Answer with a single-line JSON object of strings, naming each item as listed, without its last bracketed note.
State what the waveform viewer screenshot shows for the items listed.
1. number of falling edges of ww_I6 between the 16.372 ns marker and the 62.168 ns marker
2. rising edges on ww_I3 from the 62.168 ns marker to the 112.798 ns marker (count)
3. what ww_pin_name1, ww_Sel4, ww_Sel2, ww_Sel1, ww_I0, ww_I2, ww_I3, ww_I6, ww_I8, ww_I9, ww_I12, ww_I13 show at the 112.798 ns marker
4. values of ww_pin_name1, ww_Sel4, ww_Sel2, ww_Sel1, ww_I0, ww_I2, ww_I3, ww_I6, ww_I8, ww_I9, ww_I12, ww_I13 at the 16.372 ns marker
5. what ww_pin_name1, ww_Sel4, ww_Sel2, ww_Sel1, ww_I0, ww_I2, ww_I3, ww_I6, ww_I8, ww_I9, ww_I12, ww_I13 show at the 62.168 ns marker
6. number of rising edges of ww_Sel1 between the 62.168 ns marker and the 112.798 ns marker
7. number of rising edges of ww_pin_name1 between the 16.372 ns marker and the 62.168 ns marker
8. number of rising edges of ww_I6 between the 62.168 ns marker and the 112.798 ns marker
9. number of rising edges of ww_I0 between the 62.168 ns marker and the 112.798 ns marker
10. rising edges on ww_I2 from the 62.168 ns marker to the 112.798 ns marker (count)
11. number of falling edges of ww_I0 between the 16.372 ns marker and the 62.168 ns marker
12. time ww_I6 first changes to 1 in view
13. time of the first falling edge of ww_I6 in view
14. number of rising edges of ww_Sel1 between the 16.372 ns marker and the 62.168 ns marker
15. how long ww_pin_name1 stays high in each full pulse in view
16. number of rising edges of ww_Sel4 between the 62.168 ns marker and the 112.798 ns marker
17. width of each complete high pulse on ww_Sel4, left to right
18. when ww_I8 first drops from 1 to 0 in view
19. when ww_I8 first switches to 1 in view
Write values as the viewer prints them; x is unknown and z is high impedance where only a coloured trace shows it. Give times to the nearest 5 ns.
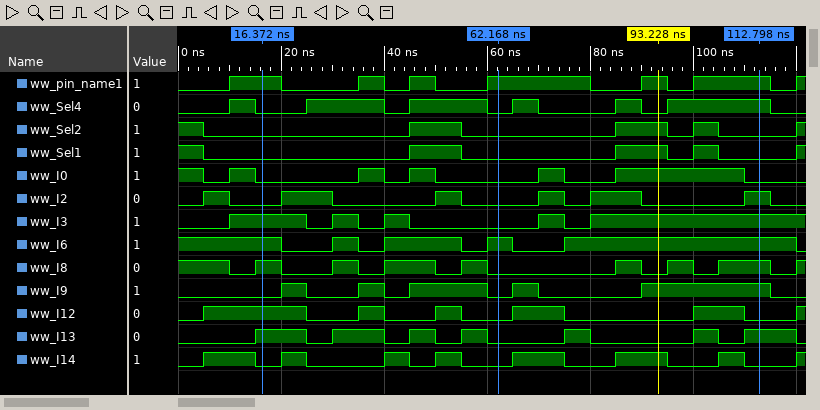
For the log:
{"number of falling edges of ww_I6 between the 16.372 ns marker and the 62.168 ns marker": "3", "rising edges on ww_I3 from the 62.168 ns marker to the 112.798 ns marker": "2", "what ww_pin_name1, ww_Sel4, ww_Sel2, ww_Sel1, ww_I0, ww_I2, ww_I3, ww_I6, ww_I8, ww_I9, ww_I12, ww_I13 show at the 112.798 ns marker": "ww_pin_name1=1, ww_Sel4=1, ww_Sel2=0, ww_Sel1=0, ww_I0=0, ww_I2=1, ww_I3=1, ww_I6=1, ww_I8=1, ww_I9=1, ww_I12=0, ww_I13=1", "values of ww_pin_name1, ww_Sel4, ww_Sel2, ww_Sel1, ww_I0, ww_I2, ww_I3, ww_I6, ww_I8, ww_I9, ww_I12, ww_I13 at the 16.372 ns marker": "ww_pin_name1=1, ww_Sel4=0, ww_Sel2=0, ww_Sel1=0, ww_I0=0, ww_I2=0, ww_I3=1, ww_I6=1, ww_I8=1, ww_I9=0, ww_I12=1, ww_I13=1", "what ww_pin_name1, ww_Sel4, ww_Sel2, ww_Sel1, ww_I0, ww_I2, ww_I3, ww_I6, ww_I8, ww_I9, ww_I12, ww_I13 show at the 62.168 ns marker": "ww_pin_name1=1, ww_Sel4=0, ww_Sel2=0, ww_Sel1=0, ww_I0=0, ww_I2=0, ww_I3=0, ww_I6=1, ww_I8=0, ww_I9=0, ww_I12=0, ww_I13=0", "number of rising edges of ww_Sel1 between the 62.168 ns marker and the 112.798 ns marker": "2", "number of rising edges of ww_pin_name1 between the 16.372 ns marker and the 62.168 ns marker": "3", "number of rising edges of ww_I6 between the 62.168 ns marker and the 112.798 ns marker": "1", "number of rising edges of ww_I0 between the 62.168 ns marker and the 112.798 ns marker": "2", "rising edges on ww_I2 from the 62.168 ns marker to the 112.798 ns marker": "3", "number of falling edges of ww_I0 between the 16.372 ns marker and the 62.168 ns marker": "2", "time ww_I6 first changes to 1 in view": "30 ns", "time of the first falling edge of ww_I6 in view": "20 ns", "number of rising edges of ww_Sel1 between the 16.372 ns marker and the 62.168 ns marker": "1", "how long ww_pin_name1 stays high in each full pulse in view": "10 ns, 5 ns, 5 ns, 20 ns, 5 ns, 15 ns", "number of rising edges of ww_Sel4 between the 62.168 ns marker and the 112.798 ns marker": "3", "width of each complete high pulse on ww_Sel4, left to right": "5 ns, 15 ns, 15 ns, 5 ns, 5 ns, 20 ns", "when ww_I8 first drops from 1 to 0 in view": "10 ns", "when ww_I8 first switches to 1 in view": "15 ns"}
